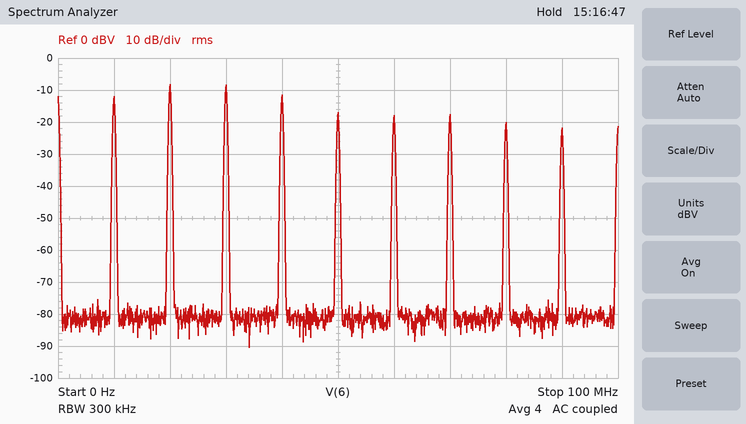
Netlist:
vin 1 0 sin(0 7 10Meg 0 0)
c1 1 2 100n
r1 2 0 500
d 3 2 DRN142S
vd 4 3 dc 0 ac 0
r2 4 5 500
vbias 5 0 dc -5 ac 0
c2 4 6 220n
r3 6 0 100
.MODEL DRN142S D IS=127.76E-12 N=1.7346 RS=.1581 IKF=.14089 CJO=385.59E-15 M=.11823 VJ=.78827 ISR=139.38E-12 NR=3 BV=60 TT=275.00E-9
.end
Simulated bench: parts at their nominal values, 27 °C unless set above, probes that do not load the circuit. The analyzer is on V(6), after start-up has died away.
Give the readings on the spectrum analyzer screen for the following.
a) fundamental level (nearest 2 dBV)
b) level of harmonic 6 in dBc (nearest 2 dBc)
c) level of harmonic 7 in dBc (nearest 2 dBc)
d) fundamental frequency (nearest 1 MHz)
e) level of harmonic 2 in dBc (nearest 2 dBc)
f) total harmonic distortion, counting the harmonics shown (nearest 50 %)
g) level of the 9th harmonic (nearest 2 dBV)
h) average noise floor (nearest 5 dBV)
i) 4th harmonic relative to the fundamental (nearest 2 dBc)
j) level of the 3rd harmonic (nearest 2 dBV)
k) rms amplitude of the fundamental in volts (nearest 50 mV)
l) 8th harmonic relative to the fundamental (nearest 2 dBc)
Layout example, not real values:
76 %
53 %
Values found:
-12 dBV
-6 dBc
-6 dBc
10 MHz
4 dBc
250 %
-22 dBV
-80 dBV
0 dBc
-8 dBV
250 mV
-8 dBc
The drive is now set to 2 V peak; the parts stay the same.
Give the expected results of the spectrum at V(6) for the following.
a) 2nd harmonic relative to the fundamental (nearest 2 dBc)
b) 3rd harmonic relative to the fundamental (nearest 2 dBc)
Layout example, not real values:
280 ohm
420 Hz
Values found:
-34 dBc
-54 dBc
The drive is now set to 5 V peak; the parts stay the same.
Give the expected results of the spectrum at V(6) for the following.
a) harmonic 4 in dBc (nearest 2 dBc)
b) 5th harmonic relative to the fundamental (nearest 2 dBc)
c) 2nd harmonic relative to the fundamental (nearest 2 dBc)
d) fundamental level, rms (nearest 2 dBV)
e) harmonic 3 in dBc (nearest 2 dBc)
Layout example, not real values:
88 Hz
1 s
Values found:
-42 dBc
-50 dBc
-24 dBc
-44 dBV
-34 dBc
